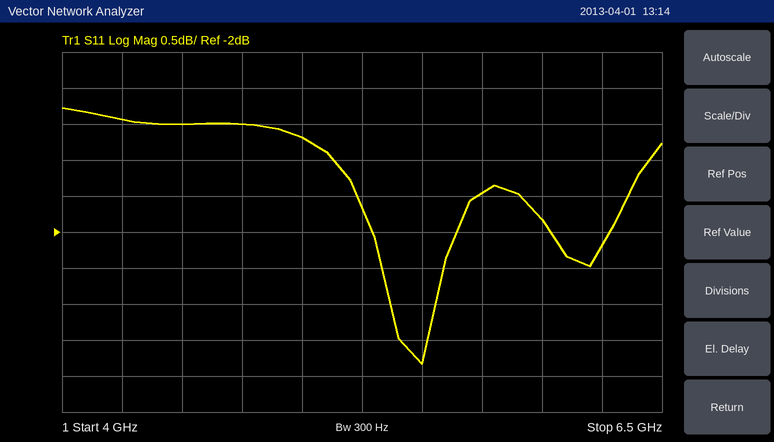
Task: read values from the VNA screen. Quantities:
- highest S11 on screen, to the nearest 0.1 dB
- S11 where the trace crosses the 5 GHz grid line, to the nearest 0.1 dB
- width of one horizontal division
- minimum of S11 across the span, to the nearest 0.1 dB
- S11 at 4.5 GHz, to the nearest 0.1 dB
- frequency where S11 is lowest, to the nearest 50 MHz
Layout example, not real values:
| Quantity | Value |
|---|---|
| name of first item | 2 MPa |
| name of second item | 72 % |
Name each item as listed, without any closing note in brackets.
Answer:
| Quantity | Value |
|---|---|
| highest S11 on screen, to the nearest 0.1 dB | -0.3 dB |
| S11 where the trace crosses the 5 GHz grid line, to the nearest 0.1 dB | -0.7 dB |
| width of one horizontal division | 250 MHz |
| minimum of S11 across the span, to the nearest 0.1 dB | -3.8 dB |
| S11 at 4.5 GHz, to the nearest 0.1 dB | -0.5 dB |
| frequency where S11 is lowest, to the nearest 50 MHz | 5.50 GHz |
